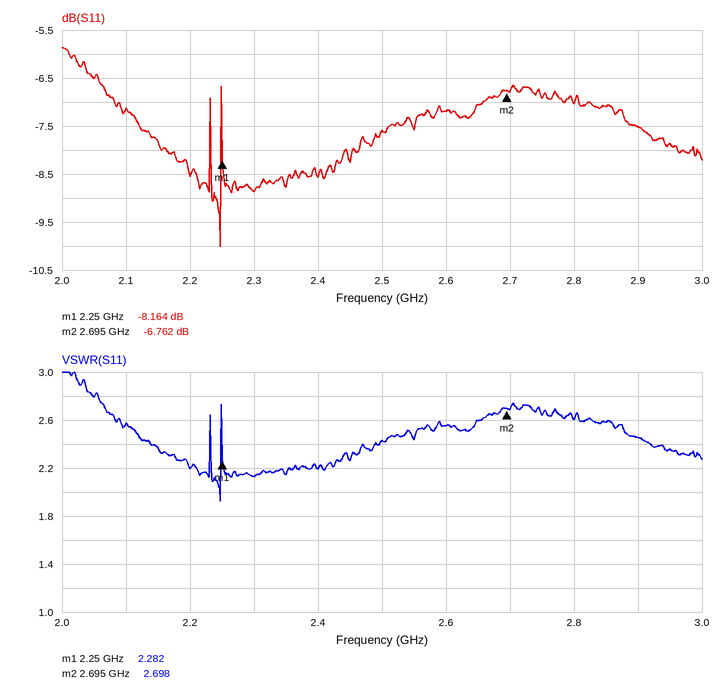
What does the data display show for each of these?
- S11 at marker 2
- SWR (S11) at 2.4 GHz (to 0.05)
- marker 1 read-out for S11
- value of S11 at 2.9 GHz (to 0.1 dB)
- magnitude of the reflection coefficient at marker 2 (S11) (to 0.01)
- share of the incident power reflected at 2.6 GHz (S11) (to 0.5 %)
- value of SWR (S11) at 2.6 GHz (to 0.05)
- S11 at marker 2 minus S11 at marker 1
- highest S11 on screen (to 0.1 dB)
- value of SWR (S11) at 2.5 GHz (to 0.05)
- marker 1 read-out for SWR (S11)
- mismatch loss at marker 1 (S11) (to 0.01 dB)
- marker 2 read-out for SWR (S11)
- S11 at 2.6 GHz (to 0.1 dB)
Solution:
-6.762 dB
2.20
-8.164 dB
-7.5 dB
0.46
19.0 %
2.55
1.402 dB
-5.9 dB
2.45
2.282
0.72 dB
2.698
-7.2 dB
